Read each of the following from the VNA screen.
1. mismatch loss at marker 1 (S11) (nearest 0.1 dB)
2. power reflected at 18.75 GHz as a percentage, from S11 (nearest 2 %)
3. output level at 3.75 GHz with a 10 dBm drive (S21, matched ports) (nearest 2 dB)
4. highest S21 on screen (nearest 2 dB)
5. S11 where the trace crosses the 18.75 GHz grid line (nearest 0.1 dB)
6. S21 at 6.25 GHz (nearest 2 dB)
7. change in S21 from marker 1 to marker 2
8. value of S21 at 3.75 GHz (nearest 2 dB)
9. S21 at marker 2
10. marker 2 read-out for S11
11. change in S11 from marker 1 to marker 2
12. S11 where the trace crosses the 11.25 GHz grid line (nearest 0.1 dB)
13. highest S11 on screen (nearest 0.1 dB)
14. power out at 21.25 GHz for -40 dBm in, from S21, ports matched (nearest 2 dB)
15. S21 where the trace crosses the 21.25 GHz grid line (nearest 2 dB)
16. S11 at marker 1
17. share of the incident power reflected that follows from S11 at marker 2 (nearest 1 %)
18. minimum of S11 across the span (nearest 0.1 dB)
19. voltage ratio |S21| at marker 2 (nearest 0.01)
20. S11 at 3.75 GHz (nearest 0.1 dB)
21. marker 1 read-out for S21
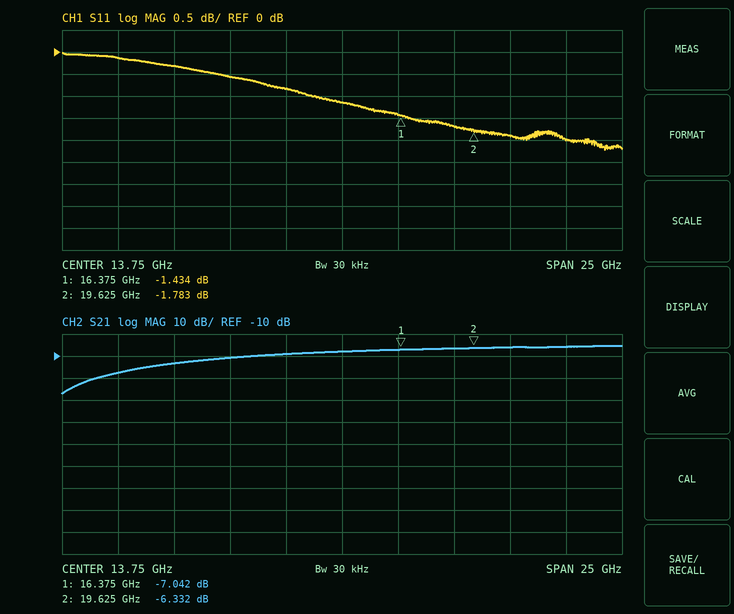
5.5 dB
68 %
-8 dBm
-6 dB
-1.7 dB
-14 dB
0.710 dB
-18 dB
-6.332 dB
-1.783 dB
-0.349 dB
-0.8 dB
0.0 dB
-46 dBm
-6 dB
-1.434 dB
66 %
-2.2 dB
0.48
-0.1 dB
-7.042 dB
